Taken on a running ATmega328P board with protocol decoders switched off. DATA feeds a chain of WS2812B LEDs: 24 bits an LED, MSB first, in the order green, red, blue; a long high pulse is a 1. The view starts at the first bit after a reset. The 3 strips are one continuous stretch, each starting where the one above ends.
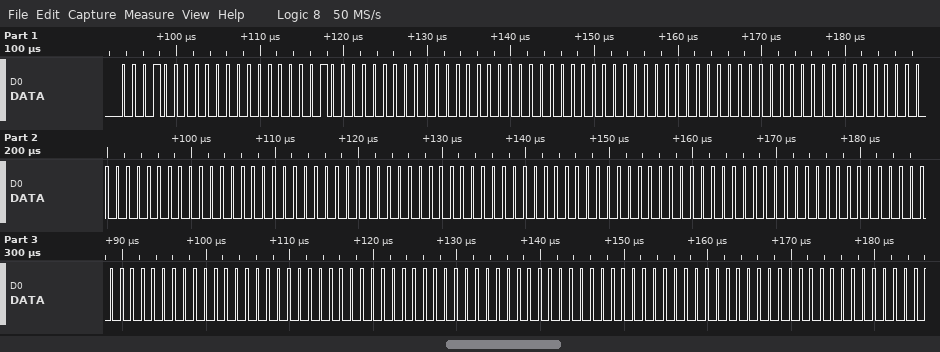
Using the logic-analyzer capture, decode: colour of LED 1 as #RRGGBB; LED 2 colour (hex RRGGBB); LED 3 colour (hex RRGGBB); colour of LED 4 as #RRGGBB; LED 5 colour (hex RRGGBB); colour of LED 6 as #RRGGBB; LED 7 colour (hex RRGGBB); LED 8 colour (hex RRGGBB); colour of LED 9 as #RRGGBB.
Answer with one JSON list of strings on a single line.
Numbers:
["#001010", "#000000", "#000000", "#000000", "#000000", "#000000", "#000000", "#000000", "#000000"]
